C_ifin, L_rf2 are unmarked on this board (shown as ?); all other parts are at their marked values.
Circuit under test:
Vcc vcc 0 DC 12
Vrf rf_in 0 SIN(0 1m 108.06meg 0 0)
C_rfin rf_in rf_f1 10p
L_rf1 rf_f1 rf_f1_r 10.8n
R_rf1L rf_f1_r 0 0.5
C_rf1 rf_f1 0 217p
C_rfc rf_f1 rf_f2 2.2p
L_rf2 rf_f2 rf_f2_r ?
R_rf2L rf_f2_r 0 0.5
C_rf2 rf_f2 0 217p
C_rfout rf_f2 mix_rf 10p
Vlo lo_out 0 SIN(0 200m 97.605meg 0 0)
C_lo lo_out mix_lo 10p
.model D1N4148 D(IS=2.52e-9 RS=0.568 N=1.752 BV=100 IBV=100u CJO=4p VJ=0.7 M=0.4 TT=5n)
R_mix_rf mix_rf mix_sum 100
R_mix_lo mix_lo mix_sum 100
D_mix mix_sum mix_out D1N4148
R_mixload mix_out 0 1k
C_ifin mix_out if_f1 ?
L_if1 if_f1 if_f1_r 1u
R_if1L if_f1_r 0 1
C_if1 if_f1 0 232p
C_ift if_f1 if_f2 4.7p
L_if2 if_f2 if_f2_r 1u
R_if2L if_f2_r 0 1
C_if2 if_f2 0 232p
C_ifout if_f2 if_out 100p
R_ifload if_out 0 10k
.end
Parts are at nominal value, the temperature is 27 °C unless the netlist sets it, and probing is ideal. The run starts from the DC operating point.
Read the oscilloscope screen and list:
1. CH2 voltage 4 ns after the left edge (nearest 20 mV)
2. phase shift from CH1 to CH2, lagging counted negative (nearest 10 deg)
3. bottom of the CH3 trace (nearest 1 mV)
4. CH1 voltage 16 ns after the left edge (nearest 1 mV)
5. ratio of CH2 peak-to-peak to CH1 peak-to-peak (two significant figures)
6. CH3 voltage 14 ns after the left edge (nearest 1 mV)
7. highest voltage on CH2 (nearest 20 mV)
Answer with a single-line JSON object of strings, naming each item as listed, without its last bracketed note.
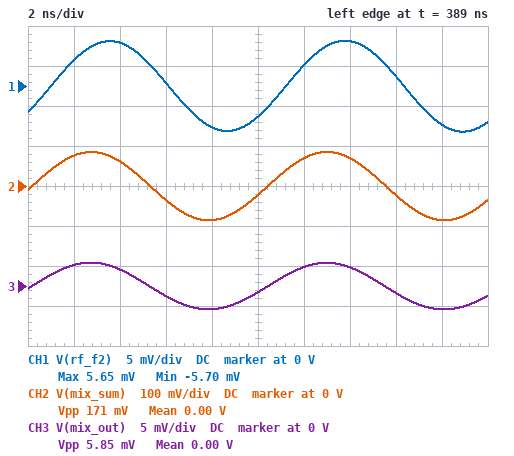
{"CH2 voltage 4 ns after the left edge": "60 mV", "phase shift from CH1 to CH2, lagging counted negative": "30 deg", "bottom of the CH3 trace": "-3 mV", "CH1 voltage 16 ns after the left edge": "1 mV", "ratio of CH2 peak-to-peak to CH1 peak-to-peak": "15", "CH3 voltage 14 ns after the left edge": "2 mV", "highest voltage on CH2": "80 mV"}
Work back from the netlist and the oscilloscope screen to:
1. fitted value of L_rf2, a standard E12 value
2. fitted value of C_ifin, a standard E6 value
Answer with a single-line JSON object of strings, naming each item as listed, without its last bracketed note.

{"fitted value of L_rf2, a standard E12 value": "27 nH", "fitted value of C_ifin, a standard E6 value": "220 pF"}
